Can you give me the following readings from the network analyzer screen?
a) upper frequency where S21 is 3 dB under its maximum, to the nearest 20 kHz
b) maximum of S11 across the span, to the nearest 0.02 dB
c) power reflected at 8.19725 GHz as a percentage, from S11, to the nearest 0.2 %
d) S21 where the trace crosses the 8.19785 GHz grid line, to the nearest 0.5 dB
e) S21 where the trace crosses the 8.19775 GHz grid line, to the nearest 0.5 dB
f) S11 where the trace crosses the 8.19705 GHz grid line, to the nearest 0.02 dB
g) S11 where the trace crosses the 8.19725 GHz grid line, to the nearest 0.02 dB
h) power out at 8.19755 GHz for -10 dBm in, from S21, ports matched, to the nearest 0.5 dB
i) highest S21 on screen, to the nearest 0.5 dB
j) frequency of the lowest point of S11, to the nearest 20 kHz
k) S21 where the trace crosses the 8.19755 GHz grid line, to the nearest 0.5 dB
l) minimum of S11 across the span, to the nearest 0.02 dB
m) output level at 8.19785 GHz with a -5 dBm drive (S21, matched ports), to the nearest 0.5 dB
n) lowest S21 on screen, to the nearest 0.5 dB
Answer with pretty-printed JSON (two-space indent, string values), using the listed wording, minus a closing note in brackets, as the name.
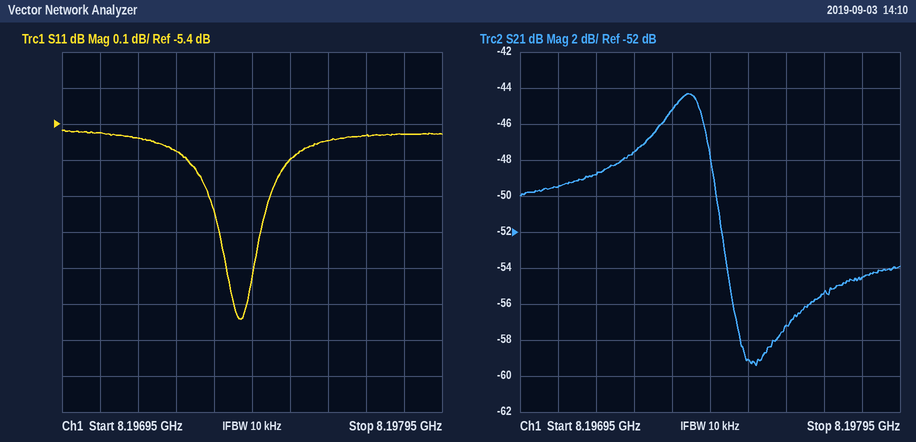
{
  "upper frequency where S21 is 3 dB under its maximum, to the nearest 20 kHz": "8.19744 GHz",
  "maximum of S11 across the span, to the nearest 0.02 dB": "-5.42 dB",
  "power reflected at 8.19725 GHz as a percentage, from S11, to the nearest 0.2 %": "28.4 %",
  "S21 where the trace crosses the 8.19785 GHz grid line, to the nearest 0.5 dB": "-54.5 dB",
  "S21 where the trace crosses the 8.19775 GHz grid line, to the nearest 0.5 dB": "-55.5 dB",
  "S11 where the trace crosses the 8.19705 GHz grid line, to the nearest 0.02 dB": "-5.42 dB",
  "S11 where the trace crosses the 8.19725 GHz grid line, to the nearest 0.02 dB": "-5.48 dB",
  "power out at 8.19755 GHz for -10 dBm in, from S21, ports matched, to the nearest 0.5 dB": "-69.0 dBm",
  "highest S21 on screen, to the nearest 0.5 dB": "-44.5 dB",
  "frequency of the lowest point of S11, to the nearest 20 kHz": "8.19742 GHz",
  "S21 where the trace crosses the 8.19755 GHz grid line, to the nearest 0.5 dB": "-59.0 dB",
  "minimum of S11 across the span, to the nearest 0.02 dB": "-5.94 dB",
  "output level at 8.19785 GHz with a -5 dBm drive (S21, matched ports), to the nearest 0.5 dB": "-59.5 dBm",
  "lowest S21 on screen, to the nearest 0.5 dB": "-59.5 dB"
}
